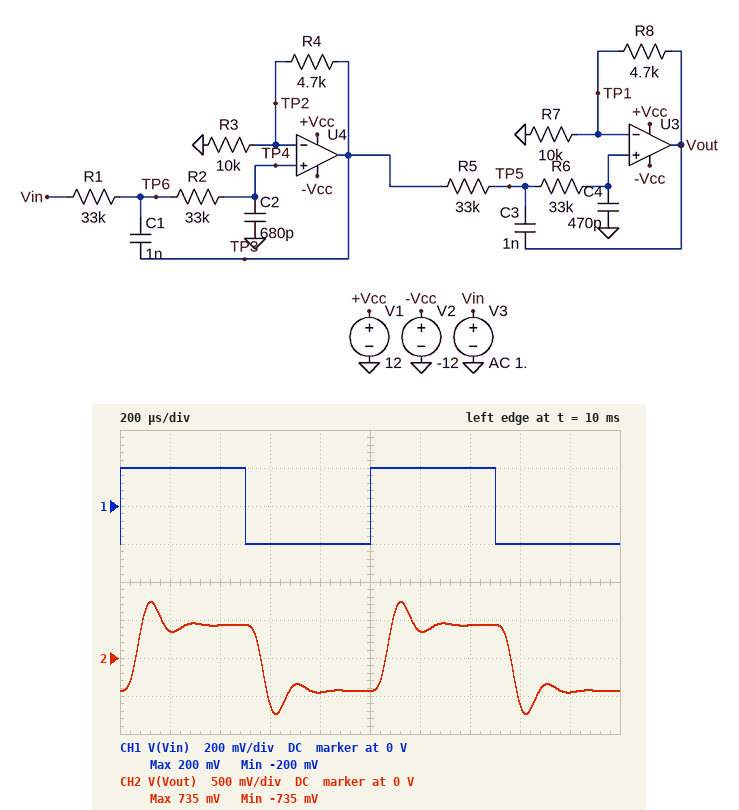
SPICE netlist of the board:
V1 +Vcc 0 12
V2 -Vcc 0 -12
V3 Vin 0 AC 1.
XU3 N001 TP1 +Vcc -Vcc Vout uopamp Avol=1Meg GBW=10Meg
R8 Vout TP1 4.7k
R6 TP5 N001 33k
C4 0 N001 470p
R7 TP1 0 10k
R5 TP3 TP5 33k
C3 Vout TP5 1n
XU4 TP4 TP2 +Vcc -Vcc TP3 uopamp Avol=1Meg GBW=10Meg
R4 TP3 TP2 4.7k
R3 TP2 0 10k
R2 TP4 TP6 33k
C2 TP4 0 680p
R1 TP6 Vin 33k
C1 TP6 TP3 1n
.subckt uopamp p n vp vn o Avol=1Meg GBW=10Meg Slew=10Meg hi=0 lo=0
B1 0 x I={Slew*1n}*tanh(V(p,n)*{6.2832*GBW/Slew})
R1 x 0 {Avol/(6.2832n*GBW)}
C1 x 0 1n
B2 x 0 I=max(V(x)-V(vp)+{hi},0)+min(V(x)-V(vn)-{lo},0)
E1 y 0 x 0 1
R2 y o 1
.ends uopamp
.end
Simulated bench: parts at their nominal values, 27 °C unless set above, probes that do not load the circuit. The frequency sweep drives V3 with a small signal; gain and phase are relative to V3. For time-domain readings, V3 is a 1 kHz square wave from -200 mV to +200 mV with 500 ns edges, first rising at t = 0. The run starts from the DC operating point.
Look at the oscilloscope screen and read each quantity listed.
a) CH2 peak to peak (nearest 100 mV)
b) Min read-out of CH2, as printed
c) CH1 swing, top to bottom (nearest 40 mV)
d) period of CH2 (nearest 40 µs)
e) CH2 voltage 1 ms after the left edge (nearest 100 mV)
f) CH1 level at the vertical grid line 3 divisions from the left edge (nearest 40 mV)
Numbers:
1.5 V
-735 mV
400 mV
1.00 ms
-400 mV
-200 mV
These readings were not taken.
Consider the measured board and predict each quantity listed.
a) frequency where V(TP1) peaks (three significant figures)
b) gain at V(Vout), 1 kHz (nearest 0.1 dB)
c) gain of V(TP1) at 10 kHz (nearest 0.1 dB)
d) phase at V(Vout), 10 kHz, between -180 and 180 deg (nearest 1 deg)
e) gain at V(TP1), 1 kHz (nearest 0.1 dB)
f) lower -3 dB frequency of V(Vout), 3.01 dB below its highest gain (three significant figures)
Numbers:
5.07 kHz
6.9 dB
-8.2 dB
87 deg
3.6 dB
1.48 kHz
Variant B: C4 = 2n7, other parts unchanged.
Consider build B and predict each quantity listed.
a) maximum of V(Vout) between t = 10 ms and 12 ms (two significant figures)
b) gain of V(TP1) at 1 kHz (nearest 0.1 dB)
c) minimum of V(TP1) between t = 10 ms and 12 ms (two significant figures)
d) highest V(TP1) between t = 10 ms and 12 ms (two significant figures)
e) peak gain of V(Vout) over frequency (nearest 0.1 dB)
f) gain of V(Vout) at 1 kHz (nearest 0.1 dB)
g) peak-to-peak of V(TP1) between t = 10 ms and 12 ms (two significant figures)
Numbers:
400 mV
0.8 dB
-270 mV
270 mV
6.7 dB
4.2 dB
540 mV
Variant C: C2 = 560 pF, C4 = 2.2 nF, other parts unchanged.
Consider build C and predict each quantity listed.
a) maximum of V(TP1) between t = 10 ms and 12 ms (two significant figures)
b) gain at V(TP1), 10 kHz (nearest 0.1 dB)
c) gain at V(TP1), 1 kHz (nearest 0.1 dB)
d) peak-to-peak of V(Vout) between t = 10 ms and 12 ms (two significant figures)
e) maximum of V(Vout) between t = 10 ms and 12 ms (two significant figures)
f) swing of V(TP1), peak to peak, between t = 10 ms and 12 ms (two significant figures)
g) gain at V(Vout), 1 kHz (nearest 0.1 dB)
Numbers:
290 mV
-23.9 dB
1.8 dB
840 mV
420 mV
570 mV
5.1 dB
